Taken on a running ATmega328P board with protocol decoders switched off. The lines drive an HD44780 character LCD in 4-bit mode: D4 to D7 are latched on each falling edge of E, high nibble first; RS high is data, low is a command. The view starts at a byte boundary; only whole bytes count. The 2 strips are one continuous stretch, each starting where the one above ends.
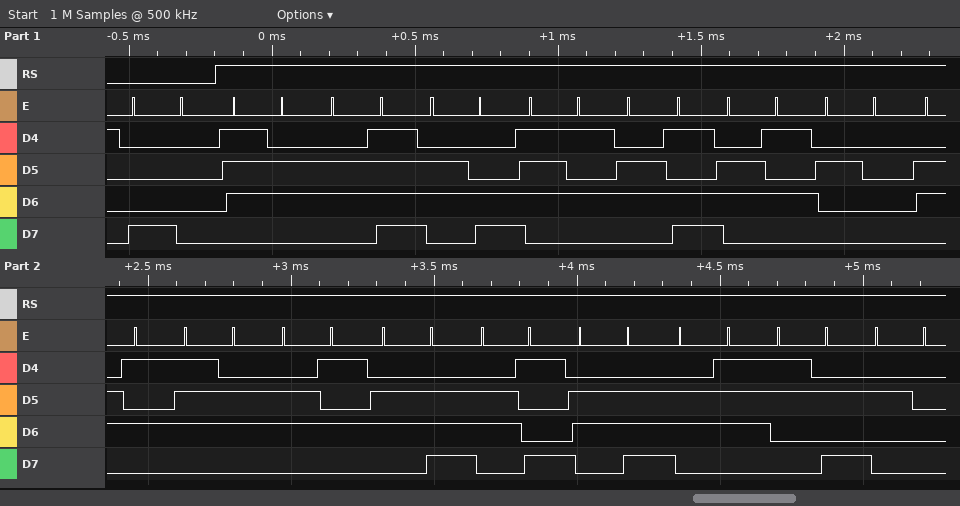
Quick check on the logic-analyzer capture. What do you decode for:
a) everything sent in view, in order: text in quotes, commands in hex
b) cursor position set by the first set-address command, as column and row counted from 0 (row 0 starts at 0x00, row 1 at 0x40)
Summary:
0x80 "volume evening: "
column 0, row 0
